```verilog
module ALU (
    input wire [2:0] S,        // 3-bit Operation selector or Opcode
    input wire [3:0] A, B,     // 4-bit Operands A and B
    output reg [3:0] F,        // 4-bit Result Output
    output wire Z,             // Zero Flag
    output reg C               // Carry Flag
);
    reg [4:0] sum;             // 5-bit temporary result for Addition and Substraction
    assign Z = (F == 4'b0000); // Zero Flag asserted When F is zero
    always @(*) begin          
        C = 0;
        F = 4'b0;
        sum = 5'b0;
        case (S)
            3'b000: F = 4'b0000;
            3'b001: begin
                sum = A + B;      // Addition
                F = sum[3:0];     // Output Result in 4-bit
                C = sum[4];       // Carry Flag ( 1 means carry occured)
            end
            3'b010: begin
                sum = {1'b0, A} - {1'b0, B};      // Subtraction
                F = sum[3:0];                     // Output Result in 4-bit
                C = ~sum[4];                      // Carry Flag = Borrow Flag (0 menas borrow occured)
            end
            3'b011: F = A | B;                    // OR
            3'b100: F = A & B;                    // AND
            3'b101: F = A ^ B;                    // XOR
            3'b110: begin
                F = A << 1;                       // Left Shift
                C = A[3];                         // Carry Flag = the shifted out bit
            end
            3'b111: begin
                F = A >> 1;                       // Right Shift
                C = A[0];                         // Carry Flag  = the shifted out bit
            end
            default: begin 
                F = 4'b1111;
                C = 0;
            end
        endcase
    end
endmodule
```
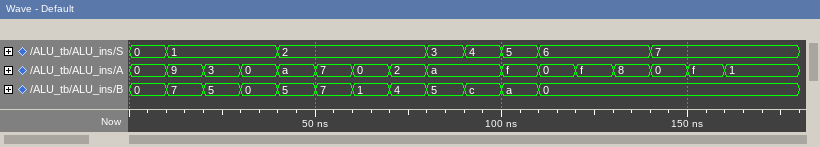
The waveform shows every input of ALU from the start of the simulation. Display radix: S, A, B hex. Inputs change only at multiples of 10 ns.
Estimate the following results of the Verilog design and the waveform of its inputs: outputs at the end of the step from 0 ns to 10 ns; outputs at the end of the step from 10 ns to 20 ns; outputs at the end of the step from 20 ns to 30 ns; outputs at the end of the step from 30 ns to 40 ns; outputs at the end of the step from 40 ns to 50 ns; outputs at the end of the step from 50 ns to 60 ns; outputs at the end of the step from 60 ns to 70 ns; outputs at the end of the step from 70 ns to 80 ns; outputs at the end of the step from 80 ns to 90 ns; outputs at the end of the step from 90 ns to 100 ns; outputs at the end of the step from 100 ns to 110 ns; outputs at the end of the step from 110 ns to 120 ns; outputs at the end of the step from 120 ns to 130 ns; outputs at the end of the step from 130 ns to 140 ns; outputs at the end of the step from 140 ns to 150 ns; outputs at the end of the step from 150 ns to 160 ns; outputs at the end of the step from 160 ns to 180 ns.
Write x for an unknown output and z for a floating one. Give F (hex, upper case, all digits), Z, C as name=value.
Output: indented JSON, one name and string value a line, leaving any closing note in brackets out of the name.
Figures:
{
  "outputs at the end of the step from 0 ns to 10 ns": "F=0, Z=1, C=0",
  "outputs at the end of the step from 10 ns to 20 ns": "F=0, Z=1, C=1",
  "outputs at the end of the step from 20 ns to 30 ns": "F=8, Z=0, C=0",
  "outputs at the end of the step from 30 ns to 40 ns": "F=0, Z=1, C=0",
  "outputs at the end of the step from 40 ns to 50 ns": "F=5, Z=0, C=1",
  "outputs at the end of the step from 50 ns to 60 ns": "F=0, Z=1, C=1",
  "outputs at the end of the step from 60 ns to 70 ns": "F=F, Z=0, C=0",
  "outputs at the end of the step from 70 ns to 80 ns": "F=E, Z=0, C=0",
  "outputs at the end of the step from 80 ns to 90 ns": "F=F, Z=0, C=0",
  "outputs at the end of the step from 90 ns to 100 ns": "F=8, Z=0, C=0",
  "outputs at the end of the step from 100 ns to 110 ns": "F=5, Z=0, C=0",
  "outputs at the end of the step from 110 ns to 120 ns": "F=0, Z=1, C=0",
  "outputs at the end of the step from 120 ns to 130 ns": "F=E, Z=0, C=1",
  "outputs at the end of the step from 130 ns to 140 ns": "F=0, Z=1, C=1",
  "outputs at the end of the step from 140 ns to 150 ns": "F=0, Z=1, C=0",
  "outputs at the end of the step from 150 ns to 160 ns": "F=7, Z=0, C=1",
  "outputs at the end of the step from 160 ns to 180 ns": "F=0, Z=1, C=1"
}
